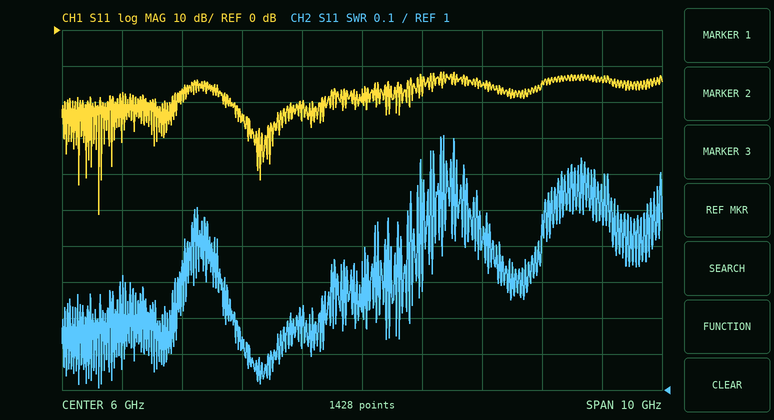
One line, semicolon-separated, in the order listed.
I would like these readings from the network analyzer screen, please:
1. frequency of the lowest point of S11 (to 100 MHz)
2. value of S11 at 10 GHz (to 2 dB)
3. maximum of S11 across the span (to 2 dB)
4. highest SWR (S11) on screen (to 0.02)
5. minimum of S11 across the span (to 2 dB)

1.6 GHz; -14 dB; -12 dB; 1.70; -52 dB
